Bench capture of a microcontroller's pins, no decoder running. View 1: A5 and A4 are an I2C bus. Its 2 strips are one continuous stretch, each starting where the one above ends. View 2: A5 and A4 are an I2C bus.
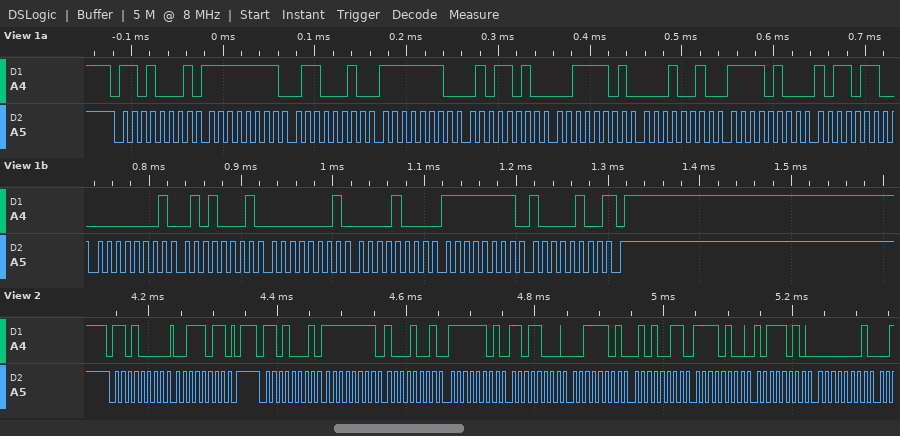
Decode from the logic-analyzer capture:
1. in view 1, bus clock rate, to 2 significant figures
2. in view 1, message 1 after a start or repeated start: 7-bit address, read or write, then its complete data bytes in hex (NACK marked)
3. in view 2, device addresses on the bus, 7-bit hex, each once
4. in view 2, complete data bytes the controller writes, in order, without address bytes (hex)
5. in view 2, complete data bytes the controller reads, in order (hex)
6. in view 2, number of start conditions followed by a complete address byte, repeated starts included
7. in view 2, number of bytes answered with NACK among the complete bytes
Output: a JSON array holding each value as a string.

["100 kHz", "0x68 read: FF 62 FE 5A 3D 12 F4 B6 01 51 01 08 FF 84 NACK", "0x68", "3B", "FF 89 FD D8 3D 53 F4 BA 01", "2", "0"]
